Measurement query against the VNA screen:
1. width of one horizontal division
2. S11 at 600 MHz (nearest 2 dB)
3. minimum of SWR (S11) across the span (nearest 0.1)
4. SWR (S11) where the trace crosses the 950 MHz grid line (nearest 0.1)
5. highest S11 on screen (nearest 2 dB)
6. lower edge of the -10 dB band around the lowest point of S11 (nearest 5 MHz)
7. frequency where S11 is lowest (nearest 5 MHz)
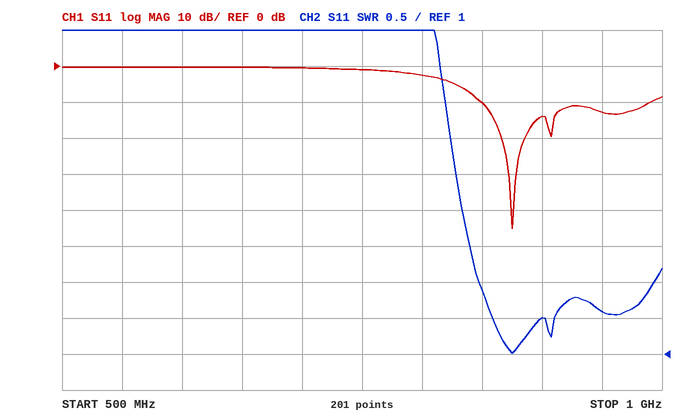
50 MHz
0 dB
1.0
1.6
0 dB
850 MHz
875 MHz
